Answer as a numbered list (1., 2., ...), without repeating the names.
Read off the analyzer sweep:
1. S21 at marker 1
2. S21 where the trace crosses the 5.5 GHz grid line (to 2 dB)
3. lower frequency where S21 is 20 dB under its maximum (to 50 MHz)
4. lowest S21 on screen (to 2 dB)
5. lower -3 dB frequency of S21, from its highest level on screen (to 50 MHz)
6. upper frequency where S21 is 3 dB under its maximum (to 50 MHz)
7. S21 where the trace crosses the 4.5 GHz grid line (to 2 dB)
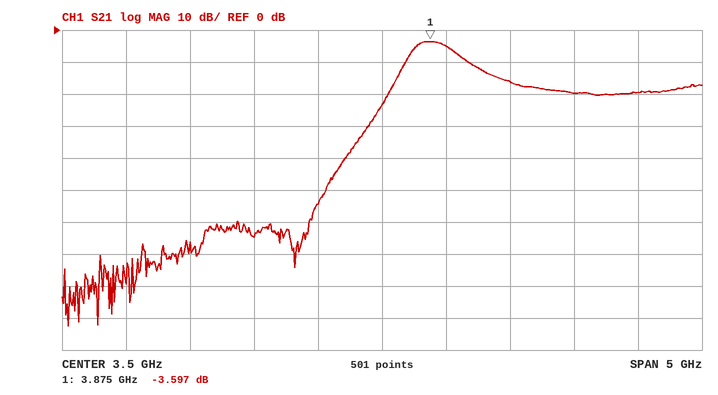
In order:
1. -3.597 dB
2. -20 dB
3. 3.50 GHz
4. -92 dB
5. 3.75 GHz
6. 4.05 GHz
7. -16 dB
